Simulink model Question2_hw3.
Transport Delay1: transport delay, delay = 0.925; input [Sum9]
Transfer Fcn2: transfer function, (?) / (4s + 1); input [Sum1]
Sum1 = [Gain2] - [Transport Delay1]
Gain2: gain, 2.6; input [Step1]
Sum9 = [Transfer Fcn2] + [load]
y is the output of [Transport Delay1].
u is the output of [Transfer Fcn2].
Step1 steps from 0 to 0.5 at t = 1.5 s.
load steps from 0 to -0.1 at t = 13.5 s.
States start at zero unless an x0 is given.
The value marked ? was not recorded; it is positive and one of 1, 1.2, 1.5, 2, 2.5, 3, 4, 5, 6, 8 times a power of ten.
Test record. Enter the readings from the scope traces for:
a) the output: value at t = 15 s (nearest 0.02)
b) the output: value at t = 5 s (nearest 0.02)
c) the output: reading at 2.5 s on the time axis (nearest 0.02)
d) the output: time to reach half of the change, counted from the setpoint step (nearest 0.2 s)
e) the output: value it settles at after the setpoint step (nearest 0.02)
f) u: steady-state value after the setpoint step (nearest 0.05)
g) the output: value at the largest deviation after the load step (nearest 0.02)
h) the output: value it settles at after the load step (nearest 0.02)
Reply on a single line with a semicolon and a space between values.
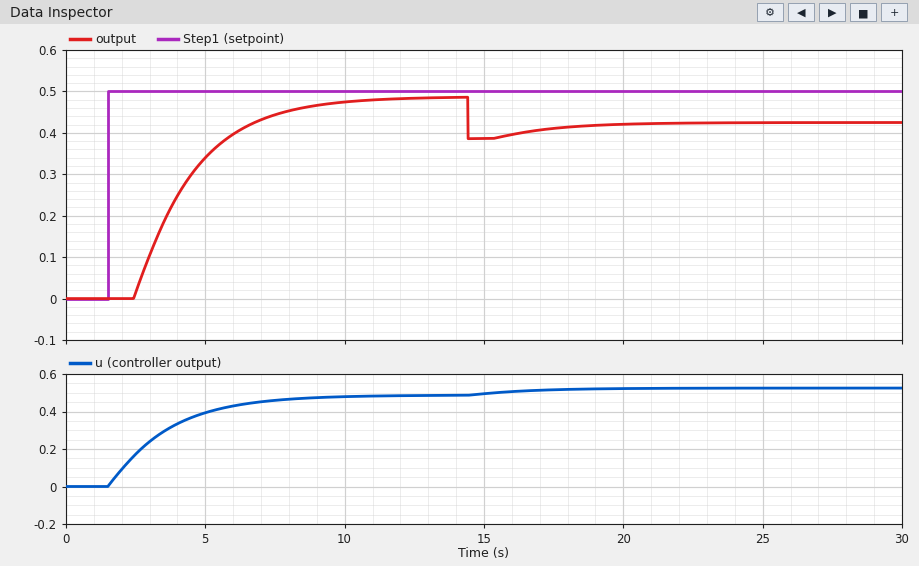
0.38; 0.34; 0.02; 2.4 s; 0.48; 0.50; 0.38; 0.42
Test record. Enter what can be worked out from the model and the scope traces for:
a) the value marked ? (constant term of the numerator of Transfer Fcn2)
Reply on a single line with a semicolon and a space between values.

0.6
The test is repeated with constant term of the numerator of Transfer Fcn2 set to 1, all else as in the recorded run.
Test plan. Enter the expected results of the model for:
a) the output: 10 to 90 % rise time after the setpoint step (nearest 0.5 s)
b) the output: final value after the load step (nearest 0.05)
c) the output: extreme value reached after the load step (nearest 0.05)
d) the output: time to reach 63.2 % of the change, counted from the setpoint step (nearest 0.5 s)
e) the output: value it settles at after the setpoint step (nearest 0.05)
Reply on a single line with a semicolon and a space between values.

3.0 s; 0.60; 0.55; 2.5 s; 0.65
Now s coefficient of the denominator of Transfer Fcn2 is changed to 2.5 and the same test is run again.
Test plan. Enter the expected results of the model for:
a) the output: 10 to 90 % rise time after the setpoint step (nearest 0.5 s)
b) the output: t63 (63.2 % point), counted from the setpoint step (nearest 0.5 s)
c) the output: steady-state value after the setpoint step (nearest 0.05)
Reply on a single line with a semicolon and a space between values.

2.5 s; 2.0 s; 0.50
